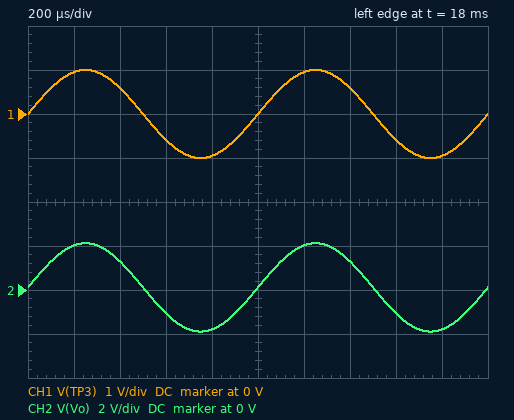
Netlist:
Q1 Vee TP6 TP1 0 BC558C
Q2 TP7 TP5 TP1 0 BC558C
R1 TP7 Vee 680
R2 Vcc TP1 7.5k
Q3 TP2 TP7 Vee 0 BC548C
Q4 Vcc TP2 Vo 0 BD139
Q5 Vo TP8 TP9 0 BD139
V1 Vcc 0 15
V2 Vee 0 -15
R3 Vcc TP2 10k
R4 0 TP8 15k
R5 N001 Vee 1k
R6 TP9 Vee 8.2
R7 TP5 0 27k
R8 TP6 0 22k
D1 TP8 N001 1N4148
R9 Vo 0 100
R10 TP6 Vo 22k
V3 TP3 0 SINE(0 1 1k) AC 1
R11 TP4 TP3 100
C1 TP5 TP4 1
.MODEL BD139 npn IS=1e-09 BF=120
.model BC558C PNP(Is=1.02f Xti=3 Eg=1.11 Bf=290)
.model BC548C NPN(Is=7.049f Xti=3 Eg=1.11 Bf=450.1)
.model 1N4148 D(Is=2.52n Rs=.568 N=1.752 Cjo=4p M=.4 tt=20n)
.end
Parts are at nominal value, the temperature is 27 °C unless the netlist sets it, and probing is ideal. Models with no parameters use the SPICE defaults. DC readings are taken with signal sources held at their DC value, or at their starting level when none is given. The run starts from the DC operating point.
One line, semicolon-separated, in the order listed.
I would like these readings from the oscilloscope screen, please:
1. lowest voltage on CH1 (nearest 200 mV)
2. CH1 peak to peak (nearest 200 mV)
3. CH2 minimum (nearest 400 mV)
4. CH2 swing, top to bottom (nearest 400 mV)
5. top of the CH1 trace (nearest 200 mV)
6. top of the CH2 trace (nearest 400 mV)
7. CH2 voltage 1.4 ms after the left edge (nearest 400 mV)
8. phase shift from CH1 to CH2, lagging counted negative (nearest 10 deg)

-1.0 V; 2.0 V; -2.0 V; 4.0 V; 1.0 V; 2.0 V; 1.2 V; 0 deg
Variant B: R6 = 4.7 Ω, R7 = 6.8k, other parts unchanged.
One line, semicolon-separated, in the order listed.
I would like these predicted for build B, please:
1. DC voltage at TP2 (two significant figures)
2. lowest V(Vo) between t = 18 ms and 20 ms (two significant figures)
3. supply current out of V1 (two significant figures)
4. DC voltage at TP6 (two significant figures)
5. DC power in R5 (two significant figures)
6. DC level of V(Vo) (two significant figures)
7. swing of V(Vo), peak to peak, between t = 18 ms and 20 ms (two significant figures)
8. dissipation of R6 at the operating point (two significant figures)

450 mV; -2.0 V; 79 mA; 24 mV; 92 µW; -22 mV; 4.0 V; 28 mW
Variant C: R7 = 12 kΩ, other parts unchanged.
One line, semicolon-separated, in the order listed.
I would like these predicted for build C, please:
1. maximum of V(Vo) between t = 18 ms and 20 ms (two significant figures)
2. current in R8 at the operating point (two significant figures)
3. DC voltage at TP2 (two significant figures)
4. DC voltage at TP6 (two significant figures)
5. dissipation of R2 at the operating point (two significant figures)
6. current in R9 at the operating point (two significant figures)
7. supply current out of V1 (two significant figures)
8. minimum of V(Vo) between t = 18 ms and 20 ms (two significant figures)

2.0 V; 1.9 µA; 480 mV; 42 mV; 27 mW; 150 µA; 64 mA; -2.0 V
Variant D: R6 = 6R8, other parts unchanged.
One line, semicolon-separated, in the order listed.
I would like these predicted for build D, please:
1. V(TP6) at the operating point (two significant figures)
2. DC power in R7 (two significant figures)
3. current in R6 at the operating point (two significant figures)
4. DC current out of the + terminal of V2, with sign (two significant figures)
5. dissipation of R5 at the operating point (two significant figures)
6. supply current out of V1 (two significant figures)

92 mV; 300 nW; 67 mA; -70 mA; 150 µW; 71 mA
